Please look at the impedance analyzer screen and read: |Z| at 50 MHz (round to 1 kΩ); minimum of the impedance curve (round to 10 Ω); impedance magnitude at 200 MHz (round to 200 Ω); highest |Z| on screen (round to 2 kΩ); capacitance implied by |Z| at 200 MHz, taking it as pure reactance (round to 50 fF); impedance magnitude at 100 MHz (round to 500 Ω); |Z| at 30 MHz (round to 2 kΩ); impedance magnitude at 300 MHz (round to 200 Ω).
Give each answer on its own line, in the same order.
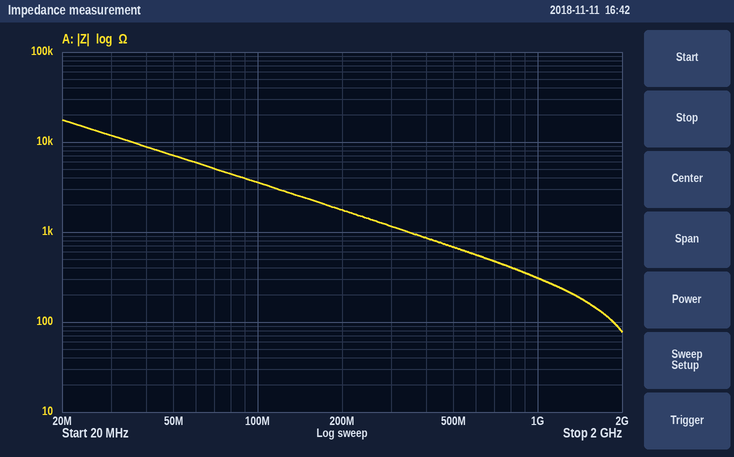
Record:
7 kΩ
80 Ω
1.8 kΩ
18 kΩ
450 fF
3.5 kΩ
12 kΩ
1.2 kΩ
